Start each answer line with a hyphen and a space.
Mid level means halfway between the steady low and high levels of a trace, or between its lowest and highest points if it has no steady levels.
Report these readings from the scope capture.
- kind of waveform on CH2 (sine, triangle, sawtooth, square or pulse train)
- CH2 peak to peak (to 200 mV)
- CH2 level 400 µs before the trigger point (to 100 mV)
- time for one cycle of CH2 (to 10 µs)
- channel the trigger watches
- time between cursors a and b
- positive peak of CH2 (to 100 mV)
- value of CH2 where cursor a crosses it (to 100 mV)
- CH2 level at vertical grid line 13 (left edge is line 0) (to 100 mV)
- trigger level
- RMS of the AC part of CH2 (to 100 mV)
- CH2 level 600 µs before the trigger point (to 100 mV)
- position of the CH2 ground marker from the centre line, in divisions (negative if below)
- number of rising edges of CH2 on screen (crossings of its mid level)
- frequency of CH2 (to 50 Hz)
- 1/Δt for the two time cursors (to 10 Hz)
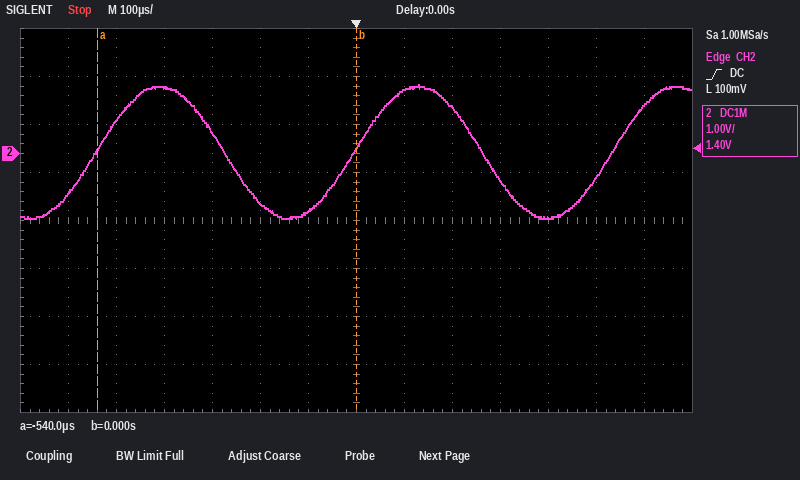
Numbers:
- sine
- 2.8 V
- 1.4 V
- 540 µs
- CH2
- 540 µs
- 1.4 V
- 100 mV
- 1.0 V
- 100 mV
- 1.0 V
- -800 mV
- +1.4 div
- 3
- 1.85 kHz
- 1.85 kHz
